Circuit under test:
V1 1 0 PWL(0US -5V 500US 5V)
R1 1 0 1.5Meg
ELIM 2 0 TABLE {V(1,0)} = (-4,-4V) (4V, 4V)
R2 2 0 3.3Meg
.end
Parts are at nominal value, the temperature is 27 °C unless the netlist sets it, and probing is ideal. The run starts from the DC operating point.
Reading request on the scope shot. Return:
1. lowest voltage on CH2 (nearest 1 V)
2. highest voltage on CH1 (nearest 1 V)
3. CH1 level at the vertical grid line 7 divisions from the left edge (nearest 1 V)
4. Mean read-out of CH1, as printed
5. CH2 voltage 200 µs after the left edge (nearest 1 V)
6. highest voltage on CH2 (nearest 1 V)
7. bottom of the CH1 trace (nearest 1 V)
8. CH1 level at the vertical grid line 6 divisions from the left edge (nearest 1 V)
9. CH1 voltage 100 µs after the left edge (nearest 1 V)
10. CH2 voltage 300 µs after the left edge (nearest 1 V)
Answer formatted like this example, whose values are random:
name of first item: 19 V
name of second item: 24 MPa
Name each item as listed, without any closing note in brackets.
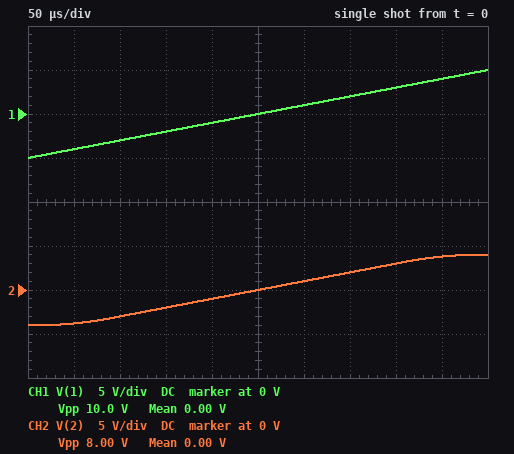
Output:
lowest voltage on CH2: -4 V
highest voltage on CH1: 5 V
CH1 level at the vertical grid line 7 divisions from the left edge: 2 V
Mean read-out of CH1, as printed: 0.00 V
CH2 voltage 200 µs after the left edge: -1 V
highest voltage on CH2: 4 V
bottom of the CH1 trace: -5 V
CH1 level at the vertical grid line 6 divisions from the left edge: 1 V
CH1 voltage 100 µs after the left edge: -3 V
CH2 voltage 300 µs after the left edge: 1 V
